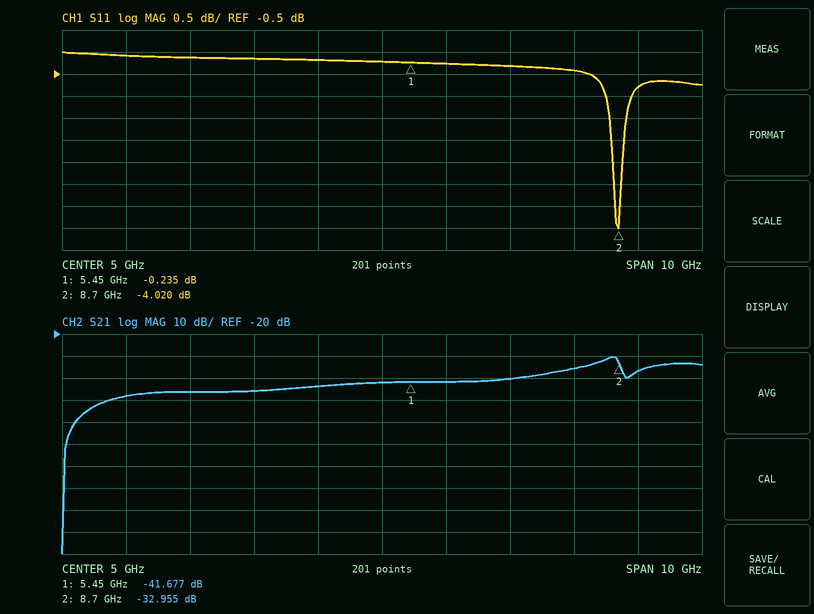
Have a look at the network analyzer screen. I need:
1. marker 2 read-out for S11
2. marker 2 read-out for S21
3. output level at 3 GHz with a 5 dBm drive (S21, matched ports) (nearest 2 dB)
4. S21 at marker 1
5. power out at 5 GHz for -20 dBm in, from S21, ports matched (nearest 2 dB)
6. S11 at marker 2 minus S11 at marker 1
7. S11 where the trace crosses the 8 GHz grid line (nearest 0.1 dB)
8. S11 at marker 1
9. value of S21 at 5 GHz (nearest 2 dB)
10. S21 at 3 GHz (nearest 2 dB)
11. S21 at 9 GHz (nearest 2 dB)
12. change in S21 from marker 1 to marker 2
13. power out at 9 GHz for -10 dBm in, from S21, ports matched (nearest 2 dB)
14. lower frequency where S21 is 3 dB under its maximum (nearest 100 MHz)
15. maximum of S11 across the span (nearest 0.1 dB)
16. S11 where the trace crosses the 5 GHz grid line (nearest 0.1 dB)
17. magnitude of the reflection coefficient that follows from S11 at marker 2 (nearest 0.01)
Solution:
-4.020 dB
-32.955 dB
-40 dBm
-41.677 dB
-62 dBm
-3.785 dB
-0.4 dB
-0.235 dB
-42 dB
-46 dB
-36 dB
8.722 dB
-46 dBm
8.3 GHz
0.0 dB
-0.2 dB
0.63
